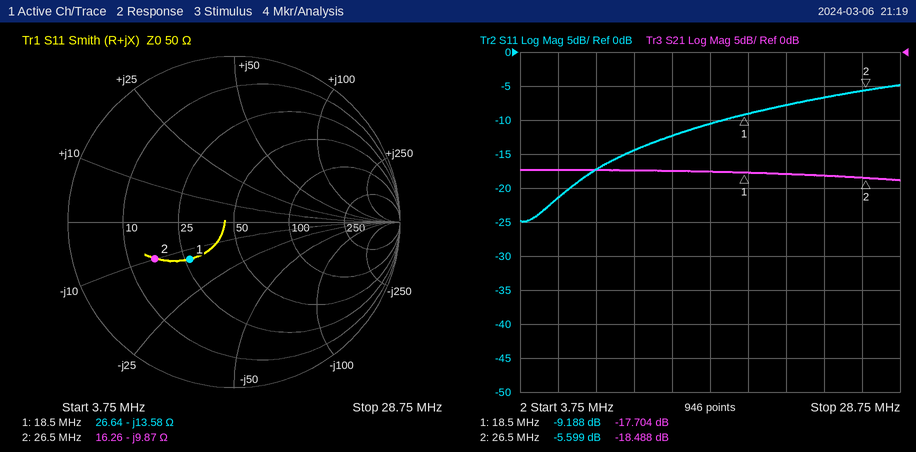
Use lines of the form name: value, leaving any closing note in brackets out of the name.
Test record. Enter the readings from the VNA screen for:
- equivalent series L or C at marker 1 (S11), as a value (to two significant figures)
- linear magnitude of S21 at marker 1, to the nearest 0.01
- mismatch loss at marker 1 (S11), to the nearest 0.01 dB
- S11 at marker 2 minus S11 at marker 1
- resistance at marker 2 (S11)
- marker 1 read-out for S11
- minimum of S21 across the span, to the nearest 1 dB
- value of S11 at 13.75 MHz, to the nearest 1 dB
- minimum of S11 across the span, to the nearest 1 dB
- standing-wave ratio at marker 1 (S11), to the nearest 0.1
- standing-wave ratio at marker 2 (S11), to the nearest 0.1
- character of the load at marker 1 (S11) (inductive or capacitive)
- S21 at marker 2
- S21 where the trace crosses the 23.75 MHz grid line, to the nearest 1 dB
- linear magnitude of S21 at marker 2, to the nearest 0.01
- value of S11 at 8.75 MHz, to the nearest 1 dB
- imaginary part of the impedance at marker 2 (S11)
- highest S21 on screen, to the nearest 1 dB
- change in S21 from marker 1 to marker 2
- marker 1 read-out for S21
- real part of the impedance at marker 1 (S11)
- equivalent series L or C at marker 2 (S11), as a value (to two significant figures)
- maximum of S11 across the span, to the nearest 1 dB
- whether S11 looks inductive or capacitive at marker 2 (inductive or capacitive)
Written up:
equivalent series L or C at marker 1 (S11), as a value: 630 pF
linear magnitude of S21 at marker 1, to the nearest 0.01: 0.13
mismatch loss at marker 1 (S11), to the nearest 0.01 dB: 0.56 dB
S11 at marker 2 minus S11 at marker 1: 3.589 dB
resistance at marker 2: 16.26 Ω
marker 1 read-out for S11: -9.188 dB
minimum of S21 across the span, to the nearest 1 dB: -19 dB
value of S11 at 13.75 MHz, to the nearest 1 dB: -12 dB
minimum of S11 across the span, to the nearest 1 dB: -25 dB
standing-wave ratio at marker 1 (S11), to the nearest 0.1: 2.1
standing-wave ratio at marker 2 (S11), to the nearest 0.1: 3.2
character of the load at marker 1 (S11): capacitive
S21 at marker 2: -18.488 dB
S21 where the trace crosses the 23.75 MHz grid line, to the nearest 1 dB: -18 dB
linear magnitude of S21 at marker 2, to the nearest 0.01: 0.12
value of S11 at 8.75 MHz, to the nearest 1 dB: -17 dB
imaginary part of the impedance at marker 2: -9.87 Ω
highest S21 on screen, to the nearest 1 dB: -17 dB
change in S21 from marker 1 to marker 2: -0.784 dB
marker 1 read-out for S21: -17.704 dB
real part of the impedance at marker 1: 26.64 Ω
equivalent series L or C at marker 2 (S11), as a value: 610 pF
maximum of S11 across the span, to the nearest 1 dB: -5 dB
whether S11 looks inductive or capacitive at marker 2: capacitive
